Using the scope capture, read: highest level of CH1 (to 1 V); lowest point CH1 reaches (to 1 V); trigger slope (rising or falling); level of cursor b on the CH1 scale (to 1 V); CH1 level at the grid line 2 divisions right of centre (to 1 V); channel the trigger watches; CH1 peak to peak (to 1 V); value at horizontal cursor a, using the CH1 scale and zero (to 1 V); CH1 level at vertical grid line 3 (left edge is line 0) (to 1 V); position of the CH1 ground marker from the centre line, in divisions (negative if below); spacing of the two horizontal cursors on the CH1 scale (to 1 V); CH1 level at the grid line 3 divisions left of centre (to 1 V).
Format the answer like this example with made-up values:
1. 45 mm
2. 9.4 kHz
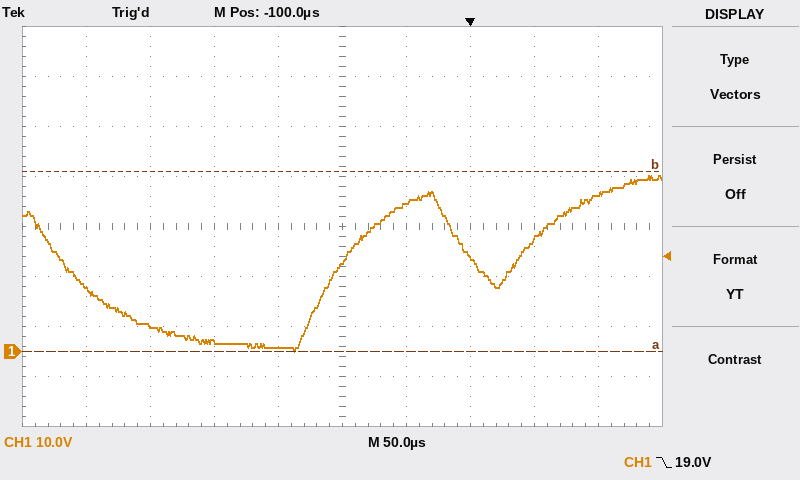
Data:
1. 35 V
2. 0 V
3. falling
4. 36 V
5. 19 V
6. CH1
7. 35 V
8. 0 V
9. 2 V
10. -2.5 div
11. 36 V
12. 5 V
